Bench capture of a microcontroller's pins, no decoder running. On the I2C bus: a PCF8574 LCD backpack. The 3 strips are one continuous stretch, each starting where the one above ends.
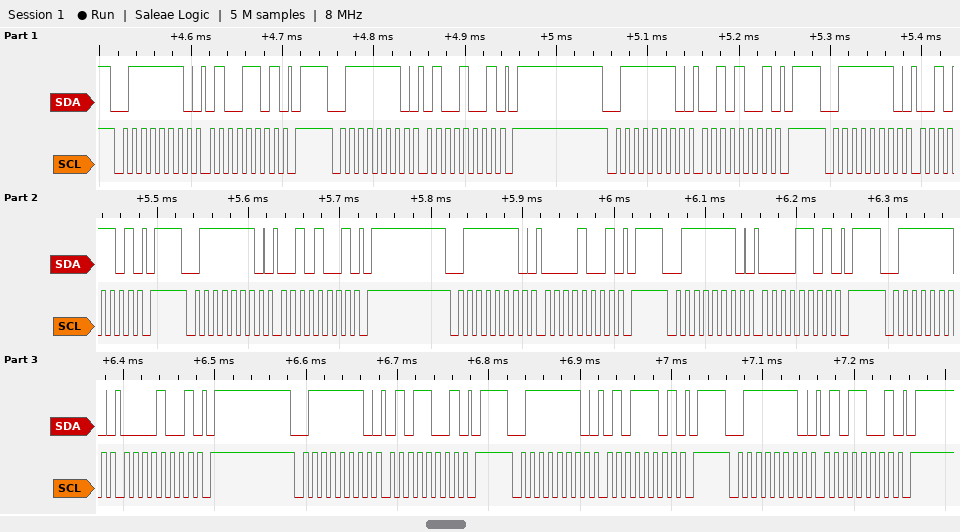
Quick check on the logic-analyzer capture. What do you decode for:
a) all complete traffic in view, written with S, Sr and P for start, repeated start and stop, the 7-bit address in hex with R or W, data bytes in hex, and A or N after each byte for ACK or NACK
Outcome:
S 3FW A 4D A P S 3FW A 49 A P S 3FW A 29 A P S 3FW A 2D A P S 3FW A 29 A P S 3FW A 09 A P S 3FW A 0D A P S 3FW A 09 A P S 3FW A 59 A P S 3FW A 5D A P S 3FW A 59 A P
